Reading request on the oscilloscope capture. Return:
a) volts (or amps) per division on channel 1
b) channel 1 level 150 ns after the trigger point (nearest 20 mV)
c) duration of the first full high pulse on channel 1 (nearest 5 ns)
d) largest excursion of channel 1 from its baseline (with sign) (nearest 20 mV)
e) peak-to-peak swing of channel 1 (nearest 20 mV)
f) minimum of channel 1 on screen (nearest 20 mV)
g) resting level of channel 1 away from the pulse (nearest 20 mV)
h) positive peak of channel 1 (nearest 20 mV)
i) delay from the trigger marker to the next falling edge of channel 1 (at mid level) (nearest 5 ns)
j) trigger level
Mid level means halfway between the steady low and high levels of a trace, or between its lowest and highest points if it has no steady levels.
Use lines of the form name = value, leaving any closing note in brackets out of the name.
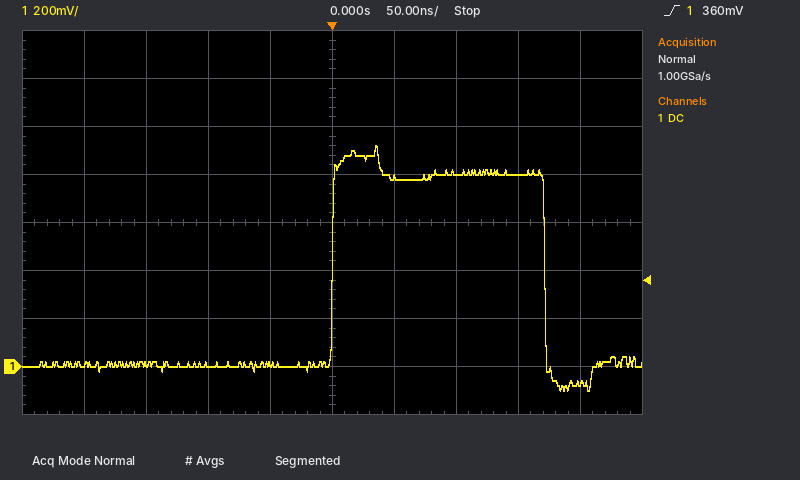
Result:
volts (or amps) per division on channel 1 = 200 mV
channel 1 level 150 ns after the trigger point = 800 mV
duration of the first full high pulse on channel 1 = 170 ns
largest excursion of channel 1 from its baseline (with sign) = +920 mV
peak-to-peak swing of channel 1 = 1.02 V
minimum of channel 1 on screen = -100 mV
resting level of channel 1 away from the pulse = 0 mV
positive peak of channel 1 = 920 mV
delay from the trigger marker to the next falling edge of channel 1 (at mid level) = 170 ns
trigger level = 360 mV
